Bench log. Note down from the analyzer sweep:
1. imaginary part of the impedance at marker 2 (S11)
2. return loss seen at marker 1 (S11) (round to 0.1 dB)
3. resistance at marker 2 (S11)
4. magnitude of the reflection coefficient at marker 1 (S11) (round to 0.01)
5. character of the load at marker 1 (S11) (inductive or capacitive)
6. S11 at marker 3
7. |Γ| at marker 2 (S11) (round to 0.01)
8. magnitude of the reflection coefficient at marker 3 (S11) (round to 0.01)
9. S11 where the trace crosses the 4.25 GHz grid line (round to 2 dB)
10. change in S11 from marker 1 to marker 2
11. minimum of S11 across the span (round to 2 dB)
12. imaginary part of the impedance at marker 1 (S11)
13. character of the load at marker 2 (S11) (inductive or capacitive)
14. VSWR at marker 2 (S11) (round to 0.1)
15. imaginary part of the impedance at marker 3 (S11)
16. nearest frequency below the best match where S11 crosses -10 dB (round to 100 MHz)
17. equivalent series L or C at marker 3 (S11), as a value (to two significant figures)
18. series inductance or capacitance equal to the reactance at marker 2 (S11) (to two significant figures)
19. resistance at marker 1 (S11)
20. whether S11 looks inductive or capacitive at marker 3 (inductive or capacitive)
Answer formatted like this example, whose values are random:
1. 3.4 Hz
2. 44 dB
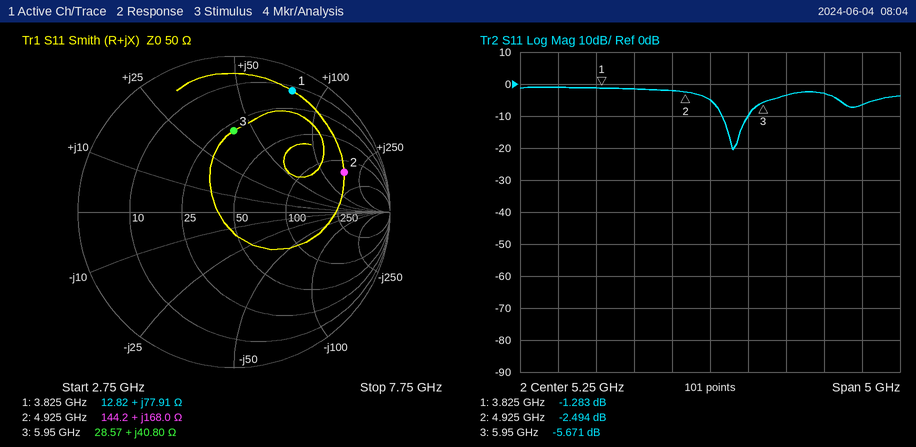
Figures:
1. +168.0 Ω
2. 1.3 dB
3. 144.2 Ω
4. 0.86
5. inductive
6. -5.671 dB
7. 0.75
8. 0.52
9. -2 dB
10. -1.211 dB
11. -20 dB
12. +77.91 Ω
13. inductive
14. 7.0
15. +40.80 Ω
16. 5.4 GHz
17. 1.1 nH
18. 5.4 nH
19. 12.82 Ω
20. inductive
